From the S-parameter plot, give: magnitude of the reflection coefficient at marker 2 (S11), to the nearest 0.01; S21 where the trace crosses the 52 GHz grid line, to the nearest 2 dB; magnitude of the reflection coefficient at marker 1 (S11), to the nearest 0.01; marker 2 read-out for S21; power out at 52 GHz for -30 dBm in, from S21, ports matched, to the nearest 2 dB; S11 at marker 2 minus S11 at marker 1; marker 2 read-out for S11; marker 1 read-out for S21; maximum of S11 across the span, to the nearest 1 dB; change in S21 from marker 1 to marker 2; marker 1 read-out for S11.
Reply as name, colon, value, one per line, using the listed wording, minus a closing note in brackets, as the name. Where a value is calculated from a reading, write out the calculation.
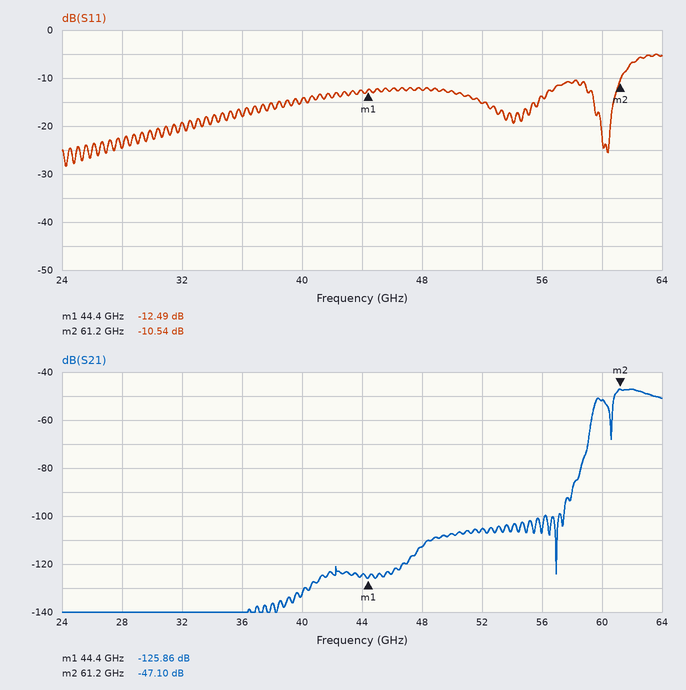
magnitude of the reflection coefficient at marker 2 (S11), to the nearest 0.01: 10^(-10.54/20) ≈ 0.30
S21 where the trace crosses the 52 GHz grid line, to the nearest 2 dB: -106 dB
magnitude of the reflection coefficient at marker 1 (S11), to the nearest 0.01: 10^(-12.49/20) ≈ 0.24
marker 2 read-out for S21: -47.10 dB
power out at 52 GHz for -30 dBm in, from S21, ports matched, to the nearest 2 dB: -30 dBm + (-106 dB) = -136 dBm
S11 at marker 2 minus S11 at marker 1: -10.54 − (-12.49) = 1.95 dB
marker 2 read-out for S11: -10.54 dB
marker 1 read-out for S21: -125.86 dB
maximum of S11 across the span, to the nearest 1 dB: -5 dB
change in S21 from marker 1 to marker 2: -47.1 − (-125.86) = 78.76 dB
marker 1 read-out for S11: -12.49 dB
